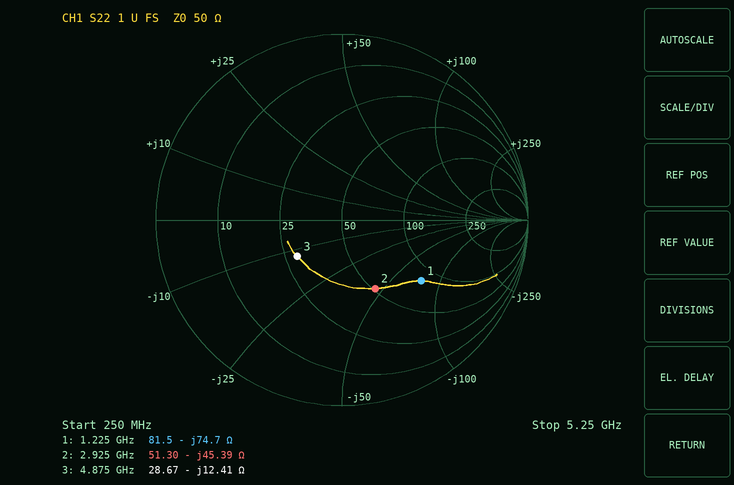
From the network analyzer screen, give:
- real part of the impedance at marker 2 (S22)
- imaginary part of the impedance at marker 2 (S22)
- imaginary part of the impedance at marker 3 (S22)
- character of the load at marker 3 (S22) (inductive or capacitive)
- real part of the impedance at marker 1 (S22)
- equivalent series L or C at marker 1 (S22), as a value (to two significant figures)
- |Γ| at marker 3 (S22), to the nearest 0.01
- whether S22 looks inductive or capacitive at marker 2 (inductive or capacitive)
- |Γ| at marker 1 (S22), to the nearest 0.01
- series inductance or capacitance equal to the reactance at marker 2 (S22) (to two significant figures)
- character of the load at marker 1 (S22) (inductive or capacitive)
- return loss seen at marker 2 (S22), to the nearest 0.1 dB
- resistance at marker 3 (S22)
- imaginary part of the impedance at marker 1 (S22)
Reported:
51.30 Ω
-45.39 Ω
-12.41 Ω
capacitive
81.5 Ω
1.7 pF
0.31
capacitive
0.54
1.2 pF
capacitive
7.8 dB
28.67 Ω
-74.7 Ω
